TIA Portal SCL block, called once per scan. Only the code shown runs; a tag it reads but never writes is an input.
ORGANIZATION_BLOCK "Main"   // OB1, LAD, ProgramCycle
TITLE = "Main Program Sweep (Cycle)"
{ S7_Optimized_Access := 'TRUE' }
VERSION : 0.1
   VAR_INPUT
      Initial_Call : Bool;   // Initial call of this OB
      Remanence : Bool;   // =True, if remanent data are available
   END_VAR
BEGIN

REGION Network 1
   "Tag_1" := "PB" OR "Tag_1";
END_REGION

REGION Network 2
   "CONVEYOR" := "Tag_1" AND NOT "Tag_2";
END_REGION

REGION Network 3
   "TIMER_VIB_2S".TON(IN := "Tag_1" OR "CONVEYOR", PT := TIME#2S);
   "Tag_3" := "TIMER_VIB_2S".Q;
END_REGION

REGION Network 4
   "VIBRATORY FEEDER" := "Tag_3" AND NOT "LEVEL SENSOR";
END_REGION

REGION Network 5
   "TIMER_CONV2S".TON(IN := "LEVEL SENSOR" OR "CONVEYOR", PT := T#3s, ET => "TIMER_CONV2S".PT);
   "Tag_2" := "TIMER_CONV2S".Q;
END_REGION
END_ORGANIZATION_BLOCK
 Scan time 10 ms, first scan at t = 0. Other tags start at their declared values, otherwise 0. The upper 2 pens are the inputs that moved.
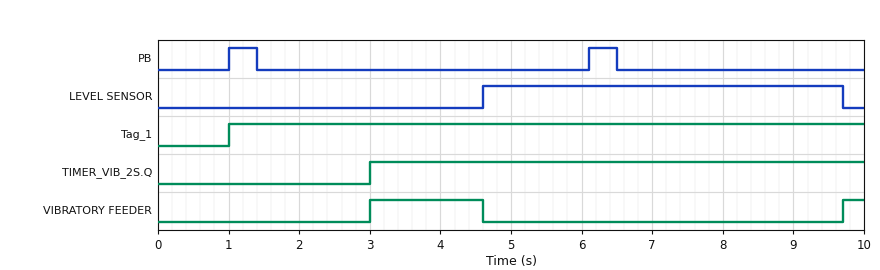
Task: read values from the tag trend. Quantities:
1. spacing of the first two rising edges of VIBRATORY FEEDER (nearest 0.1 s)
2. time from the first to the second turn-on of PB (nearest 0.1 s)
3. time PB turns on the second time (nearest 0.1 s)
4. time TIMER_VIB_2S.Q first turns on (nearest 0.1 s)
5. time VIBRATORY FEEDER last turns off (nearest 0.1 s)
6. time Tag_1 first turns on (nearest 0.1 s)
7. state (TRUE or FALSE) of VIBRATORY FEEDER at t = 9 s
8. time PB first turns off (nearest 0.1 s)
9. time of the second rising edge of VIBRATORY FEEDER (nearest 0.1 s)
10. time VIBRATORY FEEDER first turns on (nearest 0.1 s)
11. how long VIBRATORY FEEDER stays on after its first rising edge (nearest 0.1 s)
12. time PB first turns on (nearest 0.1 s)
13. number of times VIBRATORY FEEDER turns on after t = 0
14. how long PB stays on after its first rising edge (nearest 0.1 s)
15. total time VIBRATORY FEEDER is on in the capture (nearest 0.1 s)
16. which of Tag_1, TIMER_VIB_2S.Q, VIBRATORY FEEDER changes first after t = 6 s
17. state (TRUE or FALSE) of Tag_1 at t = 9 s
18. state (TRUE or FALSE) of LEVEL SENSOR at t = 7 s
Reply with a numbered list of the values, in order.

1. 6.7 s
2. 5.1 s
3. 6.1 s
4. 3.0 s
5. 4.6 s
6. 1.0 s
7. FALSE
8. 1.4 s
9. 9.7 s
10. 3.0 s
11. 1.6 s
12. 1.0 s
13. 2
14. 0.4 s
15. 1.9 s
16. VIBRATORY FEEDER
17. TRUE
18. TRUE
